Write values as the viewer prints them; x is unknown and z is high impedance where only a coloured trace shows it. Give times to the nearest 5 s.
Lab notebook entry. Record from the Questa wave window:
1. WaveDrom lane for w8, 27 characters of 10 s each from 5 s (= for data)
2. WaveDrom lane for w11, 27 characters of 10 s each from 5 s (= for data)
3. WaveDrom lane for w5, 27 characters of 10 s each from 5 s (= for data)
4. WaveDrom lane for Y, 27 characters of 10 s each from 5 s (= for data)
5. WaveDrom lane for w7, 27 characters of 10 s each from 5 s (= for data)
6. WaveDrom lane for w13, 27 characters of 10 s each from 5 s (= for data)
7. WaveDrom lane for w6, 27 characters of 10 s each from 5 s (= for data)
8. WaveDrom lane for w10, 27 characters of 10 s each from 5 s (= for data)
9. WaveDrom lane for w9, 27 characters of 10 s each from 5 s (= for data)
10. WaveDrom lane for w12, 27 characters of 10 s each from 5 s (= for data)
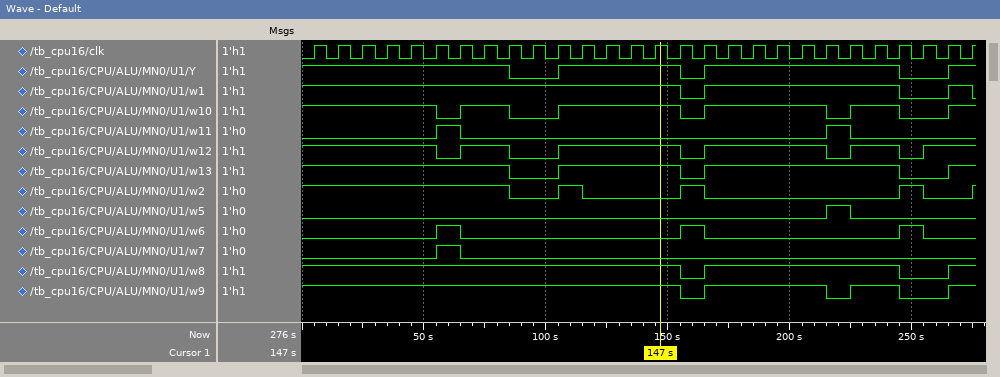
{name: 'w8', wave: '1..............01.......0.1'}
{name: 'w11', wave: '0....10..............10....'}
{name: 'w5', wave: '0....................10....'}
{name: 'Y', wave: '1.......0.1....01.......0.1'}
{name: 'w7', wave: '0....10....................'}
{name: 'w13', wave: '1.......0.1....01.......0.1'}
{name: 'w6', wave: '0....10........10.......10.'}
{name: 'w10', wave: '1....01.0.1....01....01.0.1'}
{name: 'w9', wave: '1..............01....01.0.1'}
{name: 'w12', wave: '1....01.0.1....01....01.01.'}
